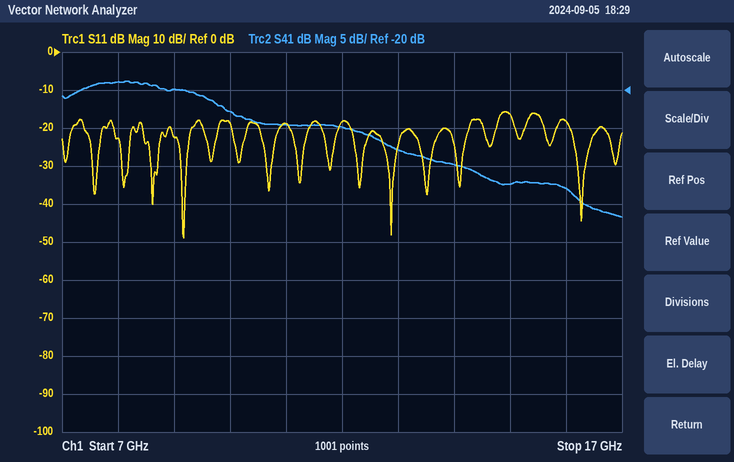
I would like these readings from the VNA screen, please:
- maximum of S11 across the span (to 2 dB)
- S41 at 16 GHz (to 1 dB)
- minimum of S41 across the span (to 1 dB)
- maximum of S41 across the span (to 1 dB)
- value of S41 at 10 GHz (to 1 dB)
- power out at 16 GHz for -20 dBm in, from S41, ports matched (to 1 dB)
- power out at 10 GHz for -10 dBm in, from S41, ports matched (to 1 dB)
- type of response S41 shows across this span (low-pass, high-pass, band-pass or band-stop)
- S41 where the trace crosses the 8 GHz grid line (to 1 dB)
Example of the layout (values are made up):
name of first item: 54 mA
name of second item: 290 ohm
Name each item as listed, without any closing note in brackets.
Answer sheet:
maximum of S11 across the span: -16 dB
S41 at 16 GHz: -33 dB
minimum of S41 across the span: -37 dB
maximum of S41 across the span: -19 dB
value of S41 at 10 GHz: -23 dB
power out at 16 GHz for -20 dBm in, from S41, ports matched: -53 dBm
power out at 10 GHz for -10 dBm in, from S41, ports matched: -33 dBm
type of response S41 shows across this span: low-pass
S41 where the trace crosses the 8 GHz grid line: -19 dB
